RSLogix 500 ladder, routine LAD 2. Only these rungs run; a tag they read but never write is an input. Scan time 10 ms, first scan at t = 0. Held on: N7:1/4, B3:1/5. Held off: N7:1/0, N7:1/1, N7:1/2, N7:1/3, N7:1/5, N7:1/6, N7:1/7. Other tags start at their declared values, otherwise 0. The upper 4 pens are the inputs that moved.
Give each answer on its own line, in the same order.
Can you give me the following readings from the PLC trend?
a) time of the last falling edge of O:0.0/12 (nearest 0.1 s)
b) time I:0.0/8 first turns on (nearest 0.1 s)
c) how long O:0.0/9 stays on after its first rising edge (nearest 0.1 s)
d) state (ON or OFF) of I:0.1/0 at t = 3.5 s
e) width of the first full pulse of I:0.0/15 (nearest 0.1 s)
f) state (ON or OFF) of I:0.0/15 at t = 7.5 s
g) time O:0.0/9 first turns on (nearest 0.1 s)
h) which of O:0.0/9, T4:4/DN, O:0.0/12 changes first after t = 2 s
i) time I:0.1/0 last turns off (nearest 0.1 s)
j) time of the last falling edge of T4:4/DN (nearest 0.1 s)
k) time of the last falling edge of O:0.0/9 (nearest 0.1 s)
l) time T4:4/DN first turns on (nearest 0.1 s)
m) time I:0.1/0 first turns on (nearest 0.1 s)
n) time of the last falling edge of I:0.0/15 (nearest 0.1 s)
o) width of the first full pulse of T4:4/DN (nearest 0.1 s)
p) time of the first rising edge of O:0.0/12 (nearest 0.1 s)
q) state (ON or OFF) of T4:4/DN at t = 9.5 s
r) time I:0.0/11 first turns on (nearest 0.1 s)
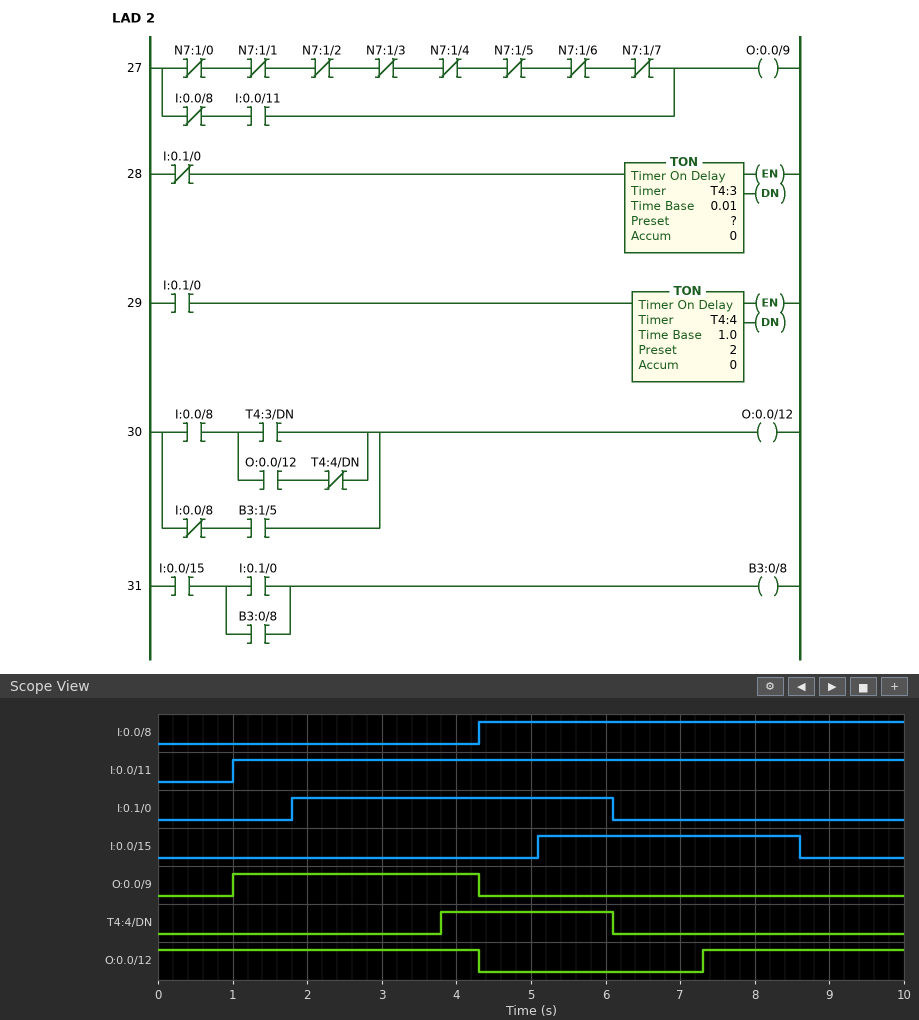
4.3 s
4.3 s
3.3 s
ON
3.5 s
ON
1.0 s
T4:4/DN
6.1 s
6.1 s
4.3 s
3.8 s
1.8 s
8.6 s
2.3 s
7.3 s
OFF
1.0 s
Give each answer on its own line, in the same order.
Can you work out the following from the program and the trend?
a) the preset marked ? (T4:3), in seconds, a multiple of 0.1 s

1.2 s
